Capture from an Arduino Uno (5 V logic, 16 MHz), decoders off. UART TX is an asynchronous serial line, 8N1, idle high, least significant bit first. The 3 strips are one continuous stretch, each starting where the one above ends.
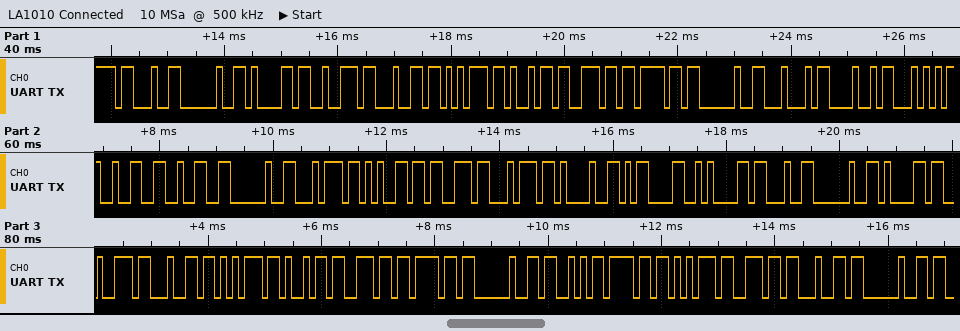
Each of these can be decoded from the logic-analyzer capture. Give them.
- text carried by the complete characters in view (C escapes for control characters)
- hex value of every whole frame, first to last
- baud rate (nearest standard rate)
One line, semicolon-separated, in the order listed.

"# arduino DHT22 test!\r\n# arduino Sound "; 23 20 61 72 64 75 69 6E 6F 20 44 48 54 32 32 20 74 65 73 74 21 0D 0A 23 20 61 72 64 75 69 6E 6F 20 53 6F 75 6E 64 20; 9600 baud
